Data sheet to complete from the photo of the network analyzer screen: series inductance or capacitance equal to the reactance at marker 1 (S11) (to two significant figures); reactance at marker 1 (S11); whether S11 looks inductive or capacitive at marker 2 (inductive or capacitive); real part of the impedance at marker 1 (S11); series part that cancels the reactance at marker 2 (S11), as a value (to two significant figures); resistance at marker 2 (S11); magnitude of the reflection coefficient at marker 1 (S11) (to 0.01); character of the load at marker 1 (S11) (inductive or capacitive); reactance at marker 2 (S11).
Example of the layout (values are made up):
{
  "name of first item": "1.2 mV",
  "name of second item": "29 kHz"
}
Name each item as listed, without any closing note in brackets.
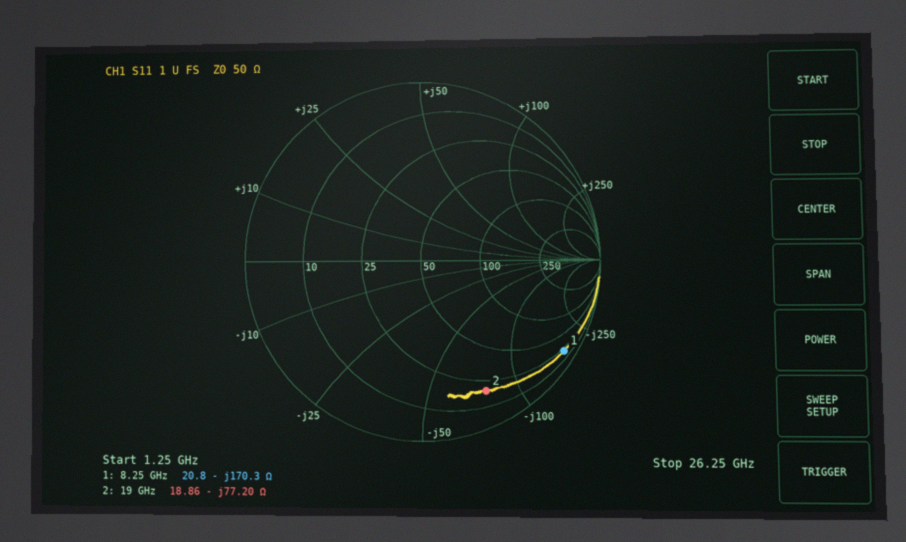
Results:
{
  "series inductance or capacitance equal to the reactance at marker 1 (S11)": "110 fF",
  "reactance at marker 1": "-170.3 Ω",
  "whether S11 looks inductive or capacitive at marker 2": "capacitive",
  "real part of the impedance at marker 1": "20.8 Ω",
  "series part that cancels the reactance at marker 2 (S11), as a value": "650 pH",
  "resistance at marker 2": "18.86 Ω",
  "magnitude of the reflection coefficient at marker 1 (S11)": "0.94",
  "character of the load at marker 1 (S11)": "capacitive",
  "reactance at marker 2": "-77.20 Ω"
}
